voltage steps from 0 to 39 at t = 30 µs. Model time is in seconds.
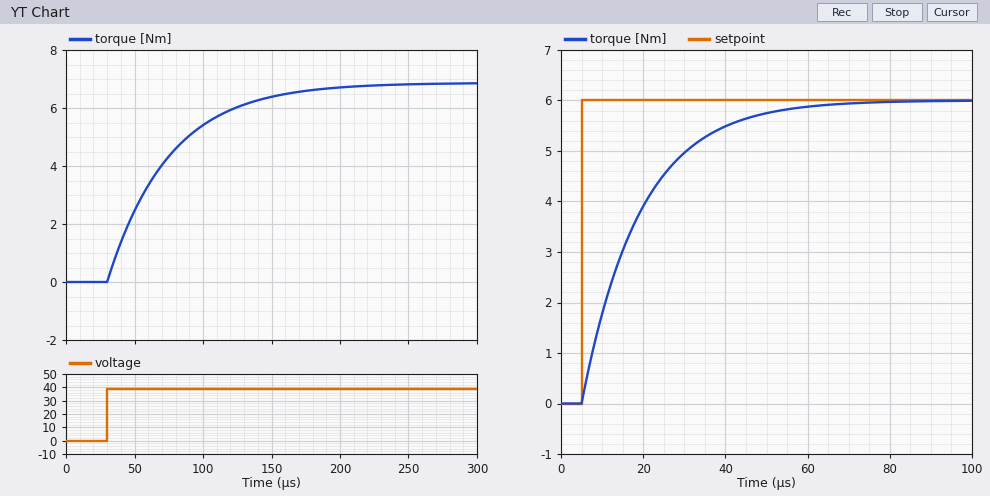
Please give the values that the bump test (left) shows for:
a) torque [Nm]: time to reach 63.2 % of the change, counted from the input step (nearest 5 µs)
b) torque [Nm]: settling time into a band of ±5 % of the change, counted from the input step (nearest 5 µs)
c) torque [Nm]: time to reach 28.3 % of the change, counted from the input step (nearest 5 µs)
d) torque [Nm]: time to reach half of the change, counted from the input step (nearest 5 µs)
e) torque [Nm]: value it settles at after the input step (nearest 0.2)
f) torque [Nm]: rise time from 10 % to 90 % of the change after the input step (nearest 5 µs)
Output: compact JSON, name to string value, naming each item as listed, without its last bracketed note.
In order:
{"torque [Nm]: time to reach 63.2 % of the change, counted from the input step": "45 µs", "torque [Nm]: settling time into a band of ±5 % of the change, counted from the input step": "135 µs", "torque [Nm]: time to reach 28.3 % of the change, counted from the input step": "15 µs", "torque [Nm]: time to reach half of the change, counted from the input step": "30 µs", "torque [Nm]: value it settles at after the input step": "6.8", "torque [Nm]: rise time from 10 % to 90 % of the change after the input step": "100 µs"}
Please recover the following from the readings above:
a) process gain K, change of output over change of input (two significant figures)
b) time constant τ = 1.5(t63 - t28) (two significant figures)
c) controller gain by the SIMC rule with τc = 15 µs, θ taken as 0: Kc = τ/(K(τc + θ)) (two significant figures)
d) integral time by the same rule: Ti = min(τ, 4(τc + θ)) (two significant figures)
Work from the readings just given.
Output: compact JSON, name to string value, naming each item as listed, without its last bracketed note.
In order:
{"process gain K, change of output over change of input": "0.17", "time constant τ = 1.5(t63 - t28)": "45 µs", "controller gain by the SIMC rule with τc = 15 µs, θ taken as 0: Kc = τ/(K(τc + θ))": "18", "integral time by the same rule: Ti = min(τ, 4(τc + θ))": "45 µs"}
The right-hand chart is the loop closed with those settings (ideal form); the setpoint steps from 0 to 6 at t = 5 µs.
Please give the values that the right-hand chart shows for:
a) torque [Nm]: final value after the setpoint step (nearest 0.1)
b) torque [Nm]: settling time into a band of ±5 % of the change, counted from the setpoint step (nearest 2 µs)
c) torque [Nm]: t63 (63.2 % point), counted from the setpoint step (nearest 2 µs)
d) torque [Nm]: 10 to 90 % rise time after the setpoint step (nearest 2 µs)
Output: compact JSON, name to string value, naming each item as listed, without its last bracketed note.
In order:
{"torque [Nm]: final value after the setpoint step": "6.0", "torque [Nm]: settling time into a band of ±5 % of the change, counted from the setpoint step": "42 µs", "torque [Nm]: t63 (63.2 % point), counted from the setpoint step": "14 µs", "torque [Nm]: 10 to 90 % rise time after the setpoint step": "32 µs"}
